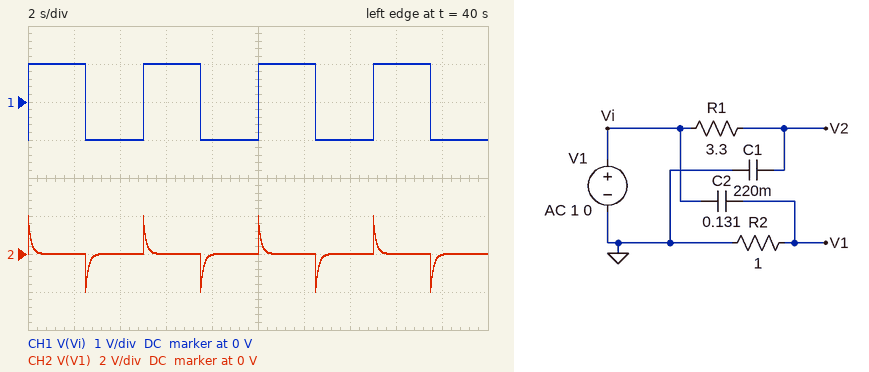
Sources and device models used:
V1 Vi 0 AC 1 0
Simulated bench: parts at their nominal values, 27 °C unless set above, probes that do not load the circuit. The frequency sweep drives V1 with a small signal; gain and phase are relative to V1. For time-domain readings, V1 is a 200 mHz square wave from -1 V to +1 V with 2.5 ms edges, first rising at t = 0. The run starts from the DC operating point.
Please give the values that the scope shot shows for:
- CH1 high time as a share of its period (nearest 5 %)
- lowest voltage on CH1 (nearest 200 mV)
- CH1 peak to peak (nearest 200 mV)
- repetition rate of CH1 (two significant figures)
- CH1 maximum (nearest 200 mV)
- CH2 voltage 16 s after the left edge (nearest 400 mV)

50 %
-1.0 V
2.0 V
200 mHz
1.0 V
0 V
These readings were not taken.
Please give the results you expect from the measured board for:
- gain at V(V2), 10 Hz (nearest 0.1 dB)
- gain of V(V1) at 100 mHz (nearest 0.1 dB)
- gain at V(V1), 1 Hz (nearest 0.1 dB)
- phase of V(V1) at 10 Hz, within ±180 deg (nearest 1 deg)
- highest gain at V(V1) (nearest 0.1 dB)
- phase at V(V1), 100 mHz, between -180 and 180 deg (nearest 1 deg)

-33.2 dB
-21.7 dB
-3.9 dB
7 deg
0 dB
85 deg
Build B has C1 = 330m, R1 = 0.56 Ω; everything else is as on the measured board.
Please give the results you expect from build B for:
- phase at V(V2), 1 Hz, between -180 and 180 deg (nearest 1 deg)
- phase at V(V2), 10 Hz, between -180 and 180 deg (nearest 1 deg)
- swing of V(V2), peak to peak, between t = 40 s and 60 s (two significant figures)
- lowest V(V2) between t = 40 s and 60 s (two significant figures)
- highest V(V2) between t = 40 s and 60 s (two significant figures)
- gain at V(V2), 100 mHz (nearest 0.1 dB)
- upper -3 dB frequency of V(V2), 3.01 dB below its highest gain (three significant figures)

-49 deg
-85 deg
2.0 V
-1.0 V
1.0 V
-0.1 dB
861 mHz
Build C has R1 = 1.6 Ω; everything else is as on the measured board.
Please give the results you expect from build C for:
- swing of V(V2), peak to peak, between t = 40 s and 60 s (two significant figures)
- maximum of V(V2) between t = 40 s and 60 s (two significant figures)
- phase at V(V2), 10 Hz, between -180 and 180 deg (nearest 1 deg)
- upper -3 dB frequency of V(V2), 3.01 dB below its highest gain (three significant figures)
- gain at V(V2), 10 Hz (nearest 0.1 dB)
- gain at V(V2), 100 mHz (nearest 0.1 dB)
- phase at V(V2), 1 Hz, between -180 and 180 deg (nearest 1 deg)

2.0 V
1.0 V
-87 deg
452 mHz
-26.9 dB
-0.2 dB
-66 deg
